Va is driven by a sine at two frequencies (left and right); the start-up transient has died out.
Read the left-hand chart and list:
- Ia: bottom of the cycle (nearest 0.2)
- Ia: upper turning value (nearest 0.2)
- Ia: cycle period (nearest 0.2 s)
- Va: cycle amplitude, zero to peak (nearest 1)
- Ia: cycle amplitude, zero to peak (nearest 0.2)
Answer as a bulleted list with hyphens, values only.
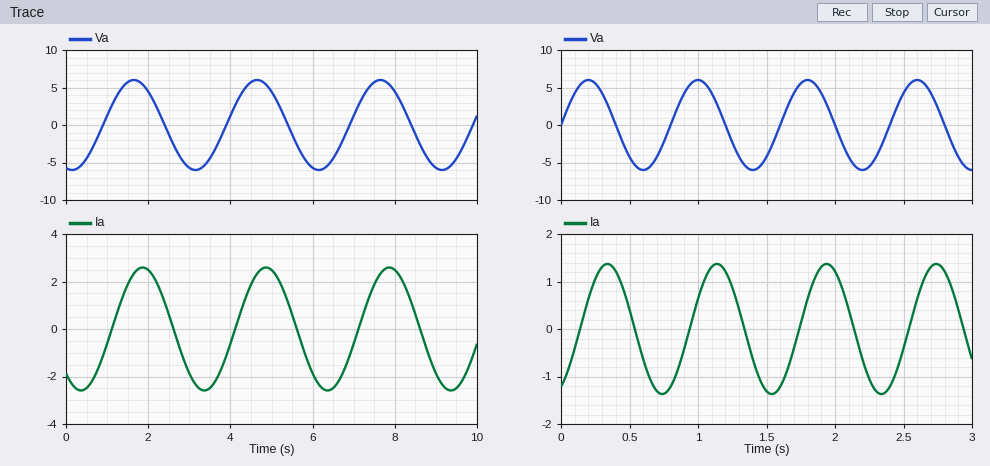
- -2.6
- 2.6
- 3.0 s
- 6
- 2.6
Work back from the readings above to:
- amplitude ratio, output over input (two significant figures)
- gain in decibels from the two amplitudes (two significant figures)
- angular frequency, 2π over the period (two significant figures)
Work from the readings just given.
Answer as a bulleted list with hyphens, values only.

- 0.43
- -7.3 dB
- 2.1 rad/s
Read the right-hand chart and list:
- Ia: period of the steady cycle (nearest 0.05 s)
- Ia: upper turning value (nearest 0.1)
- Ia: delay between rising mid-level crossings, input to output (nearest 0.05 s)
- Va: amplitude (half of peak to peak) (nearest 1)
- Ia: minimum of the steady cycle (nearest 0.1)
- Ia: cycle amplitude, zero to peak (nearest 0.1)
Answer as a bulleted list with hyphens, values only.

- 0.80 s
- 1.4
- 0.15 s
- 6
- -1.4
- 1.4
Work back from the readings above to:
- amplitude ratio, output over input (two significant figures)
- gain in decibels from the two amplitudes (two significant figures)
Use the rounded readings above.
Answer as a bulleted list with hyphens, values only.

- 0.23
- -13 dB
